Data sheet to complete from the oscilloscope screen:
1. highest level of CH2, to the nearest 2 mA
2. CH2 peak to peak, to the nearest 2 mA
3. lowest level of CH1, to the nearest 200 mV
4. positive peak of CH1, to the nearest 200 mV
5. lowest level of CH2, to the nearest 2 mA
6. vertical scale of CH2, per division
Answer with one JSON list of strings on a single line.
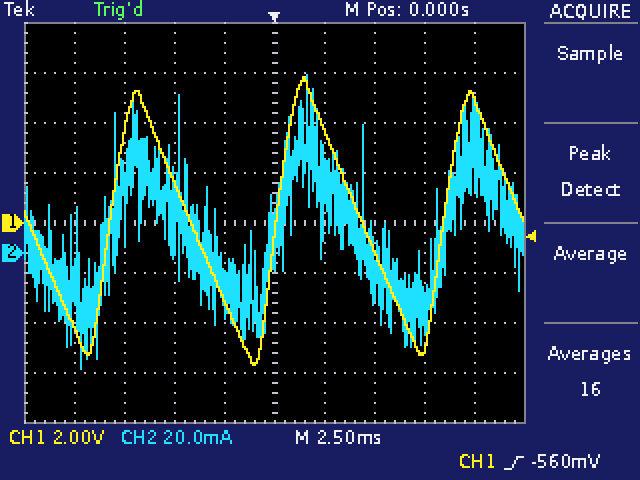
["72 mA", "118 mA", "-5.6 V", "5.8 V", "-46 mA", "20 mA"]
